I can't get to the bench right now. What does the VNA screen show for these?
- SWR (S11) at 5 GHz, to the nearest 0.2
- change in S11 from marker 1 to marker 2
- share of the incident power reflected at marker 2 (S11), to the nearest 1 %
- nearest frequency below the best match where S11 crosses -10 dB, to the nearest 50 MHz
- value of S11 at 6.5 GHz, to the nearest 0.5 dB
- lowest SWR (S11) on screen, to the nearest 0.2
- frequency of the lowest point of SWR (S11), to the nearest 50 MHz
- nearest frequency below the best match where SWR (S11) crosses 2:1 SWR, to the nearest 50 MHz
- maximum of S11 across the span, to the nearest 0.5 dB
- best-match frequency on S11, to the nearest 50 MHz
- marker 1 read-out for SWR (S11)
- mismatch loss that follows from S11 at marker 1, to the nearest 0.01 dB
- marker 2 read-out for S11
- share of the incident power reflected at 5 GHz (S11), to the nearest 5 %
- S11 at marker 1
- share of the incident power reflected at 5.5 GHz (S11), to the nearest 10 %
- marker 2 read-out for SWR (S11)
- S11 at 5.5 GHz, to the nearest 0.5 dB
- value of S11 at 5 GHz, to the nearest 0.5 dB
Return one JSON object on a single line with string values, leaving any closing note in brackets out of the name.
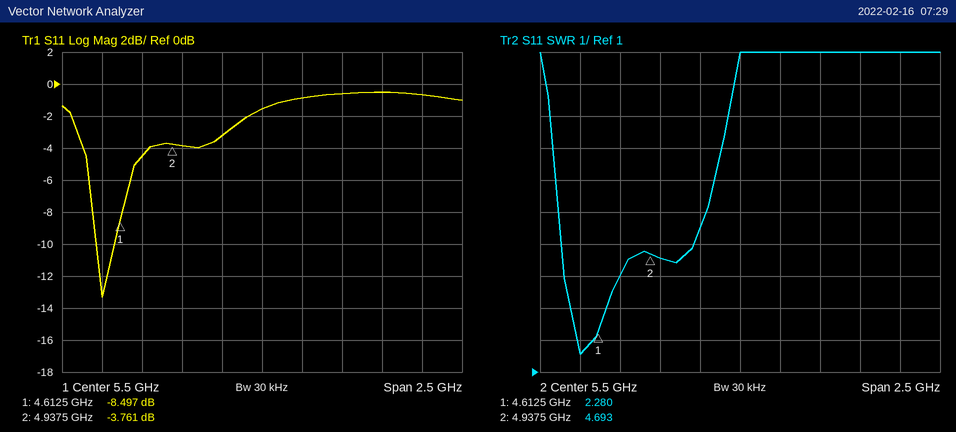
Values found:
{"SWR (S11) at 5 GHz, to the nearest 0.2": "4.6", "change in S11 from marker 1 to marker 2": "4.736 dB", "share of the incident power reflected at marker 2 (S11), to the nearest 1 %": "42 %", "nearest frequency below the best match where S11 crosses -10 dB, to the nearest 50 MHz": "4.45 GHz", "value of S11 at 6.5 GHz, to the nearest 0.5 dB": "-0.5 dB", "lowest SWR (S11) on screen, to the nearest 0.2": "1.6", "frequency of the lowest point of SWR (S11), to the nearest 50 MHz": "4.50 GHz", "nearest frequency below the best match where SWR (S11) crosses 2:1 SWR, to the nearest 50 MHz": "4.50 GHz", "maximum of S11 across the span, to the nearest 0.5 dB": "-0.5 dB", "best-match frequency on S11, to the nearest 50 MHz": "4.50 GHz", "marker 1 read-out for SWR": "2.280", "mismatch loss that follows from S11 at marker 1, to the nearest 0.01 dB": "0.66 dB", "marker 2 read-out for S11": "-3.761 dB", "share of the incident power reflected at 5 GHz (S11), to the nearest 5 %": "40 %", "S11 at marker 1": "-8.497 dB", "share of the incident power reflected at 5.5 GHz (S11), to the nearest 10 %": "70 %", "marker 2 read-out for SWR": "4.693", "S11 at 5.5 GHz, to the nearest 0.5 dB": "-1.5 dB", "value of S11 at 5 GHz, to the nearest 0.5 dB": "-4.0 dB"}
